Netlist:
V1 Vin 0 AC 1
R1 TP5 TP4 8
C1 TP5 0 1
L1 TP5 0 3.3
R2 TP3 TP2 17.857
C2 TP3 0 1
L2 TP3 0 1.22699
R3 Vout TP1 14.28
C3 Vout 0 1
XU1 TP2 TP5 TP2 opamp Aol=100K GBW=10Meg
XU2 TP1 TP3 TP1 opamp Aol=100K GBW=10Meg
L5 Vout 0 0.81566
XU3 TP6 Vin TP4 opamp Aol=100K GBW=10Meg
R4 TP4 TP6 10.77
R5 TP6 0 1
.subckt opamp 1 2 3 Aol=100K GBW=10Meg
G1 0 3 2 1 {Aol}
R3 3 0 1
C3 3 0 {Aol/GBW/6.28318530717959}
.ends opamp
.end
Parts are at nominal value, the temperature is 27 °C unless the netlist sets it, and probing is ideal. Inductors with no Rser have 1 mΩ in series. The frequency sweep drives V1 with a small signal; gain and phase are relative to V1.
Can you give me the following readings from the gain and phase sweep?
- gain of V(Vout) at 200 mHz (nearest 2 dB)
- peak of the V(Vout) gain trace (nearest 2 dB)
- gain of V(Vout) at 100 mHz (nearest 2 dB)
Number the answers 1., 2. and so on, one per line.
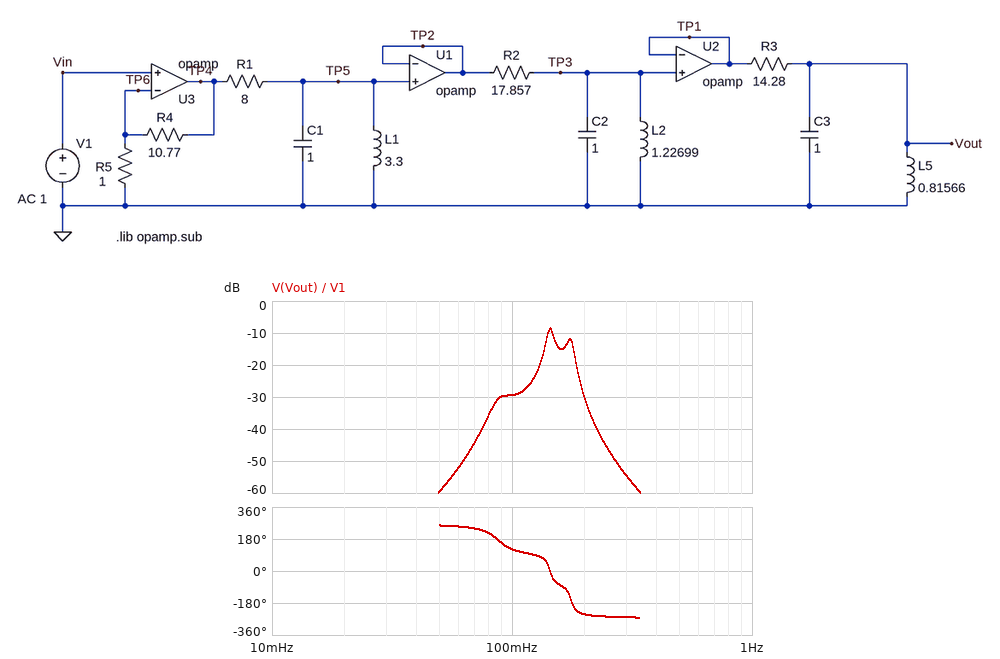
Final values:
1. -30 dB
2. -8 dB
3. -30 dB
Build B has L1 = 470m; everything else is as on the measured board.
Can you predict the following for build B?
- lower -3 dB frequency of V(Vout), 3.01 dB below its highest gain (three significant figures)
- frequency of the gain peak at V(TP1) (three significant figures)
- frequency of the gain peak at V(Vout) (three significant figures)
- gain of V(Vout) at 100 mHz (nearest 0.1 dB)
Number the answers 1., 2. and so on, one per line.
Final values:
1. 170 mHz
2. 144 mHz
3. 176 mHz
4. -52.6 dB
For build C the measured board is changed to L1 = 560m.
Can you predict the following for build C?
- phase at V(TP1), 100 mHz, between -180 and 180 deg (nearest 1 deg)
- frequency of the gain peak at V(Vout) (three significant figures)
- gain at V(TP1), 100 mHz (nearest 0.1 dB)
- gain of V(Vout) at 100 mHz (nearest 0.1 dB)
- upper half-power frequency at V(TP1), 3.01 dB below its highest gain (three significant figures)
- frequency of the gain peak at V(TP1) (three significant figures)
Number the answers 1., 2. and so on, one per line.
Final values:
1. 172 deg
2. 176 mHz
3. -25.1 dB
4. -50.7 dB
5. 149 mHz
6. 144 mHz
